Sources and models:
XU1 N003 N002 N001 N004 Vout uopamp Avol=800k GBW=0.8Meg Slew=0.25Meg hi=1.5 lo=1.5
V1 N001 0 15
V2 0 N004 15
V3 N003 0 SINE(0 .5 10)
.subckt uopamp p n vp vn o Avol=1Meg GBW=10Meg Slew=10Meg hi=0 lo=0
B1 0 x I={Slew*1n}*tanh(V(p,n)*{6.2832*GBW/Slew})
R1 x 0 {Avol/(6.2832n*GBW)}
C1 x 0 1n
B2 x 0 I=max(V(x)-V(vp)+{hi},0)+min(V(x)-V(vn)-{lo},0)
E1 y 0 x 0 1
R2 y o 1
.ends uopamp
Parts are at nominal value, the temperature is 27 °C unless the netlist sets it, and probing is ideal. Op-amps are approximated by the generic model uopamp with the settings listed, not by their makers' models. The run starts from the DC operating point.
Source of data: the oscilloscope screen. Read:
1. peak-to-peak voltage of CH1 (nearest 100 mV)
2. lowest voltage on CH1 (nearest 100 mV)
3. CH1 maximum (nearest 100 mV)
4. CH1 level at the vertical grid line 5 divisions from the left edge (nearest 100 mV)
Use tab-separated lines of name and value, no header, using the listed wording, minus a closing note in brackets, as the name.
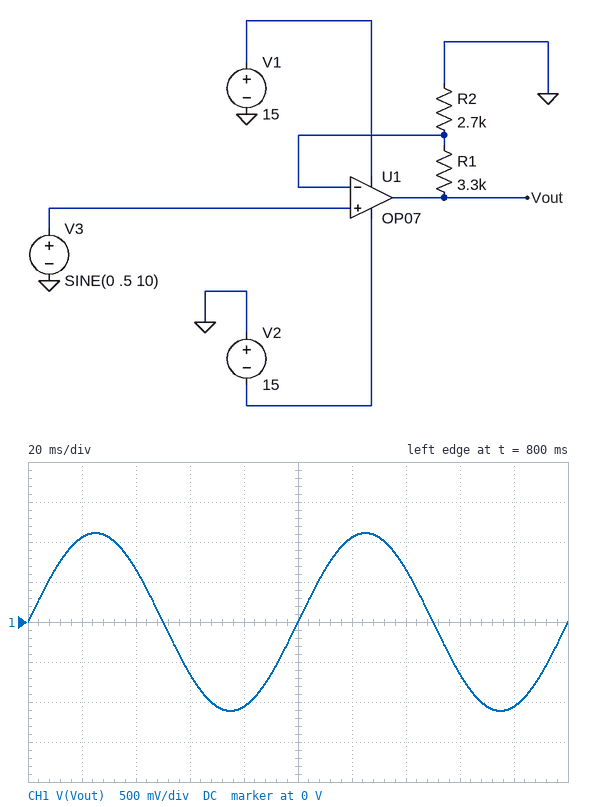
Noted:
peak-to-peak voltage of CH1	2.2 V
lowest voltage on CH1	-1.1 V
CH1 maximum	1.1 V
CH1 level at the vertical grid line 5 divisions from the left edge	0 V
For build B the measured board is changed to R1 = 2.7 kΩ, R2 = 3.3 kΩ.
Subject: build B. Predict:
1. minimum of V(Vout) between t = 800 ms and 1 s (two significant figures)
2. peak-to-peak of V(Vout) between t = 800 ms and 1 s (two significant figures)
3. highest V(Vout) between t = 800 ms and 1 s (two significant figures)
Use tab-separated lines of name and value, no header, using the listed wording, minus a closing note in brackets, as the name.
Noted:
minimum of V(Vout) between t = 800 ms and 1 s	-910 mV
peak-to-peak of V(Vout) between t = 800 ms and 1 s	1.8 V
highest V(Vout) between t = 800 ms and 1 s	910 mV
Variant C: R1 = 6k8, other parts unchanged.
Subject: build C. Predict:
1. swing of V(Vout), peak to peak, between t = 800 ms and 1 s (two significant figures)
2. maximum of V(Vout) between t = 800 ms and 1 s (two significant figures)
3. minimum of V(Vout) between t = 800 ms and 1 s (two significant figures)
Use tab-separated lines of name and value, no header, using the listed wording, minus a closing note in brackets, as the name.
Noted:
swing of V(Vout), peak to peak, between t = 800 ms and 1 s	3.5 V
maximum of V(Vout) between t = 800 ms and 1 s	1.8 V
minimum of V(Vout) between t = 800 ms and 1 s	-1.8 V
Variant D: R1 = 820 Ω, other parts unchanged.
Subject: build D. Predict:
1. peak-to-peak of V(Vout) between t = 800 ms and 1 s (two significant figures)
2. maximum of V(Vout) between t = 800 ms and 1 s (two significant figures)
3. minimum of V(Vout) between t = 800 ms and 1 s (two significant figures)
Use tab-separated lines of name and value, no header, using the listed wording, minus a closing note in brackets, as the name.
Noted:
peak-to-peak of V(Vout) between t = 800 ms and 1 s	1.3 V
maximum of V(Vout) between t = 800 ms and 1 s	650 mV
minimum of V(Vout) between t = 800 ms and 1 s	-650 mV
